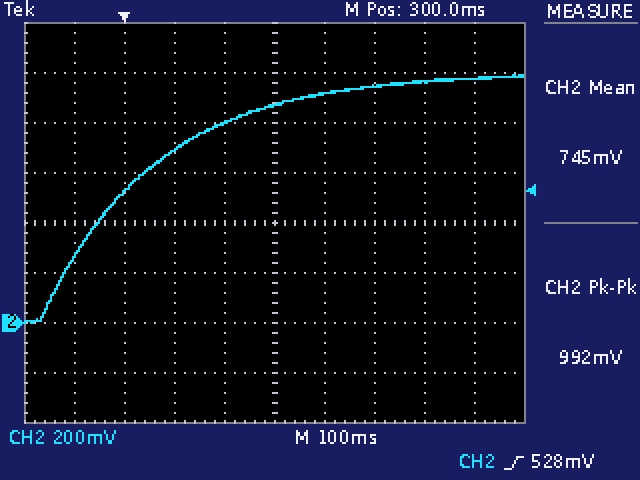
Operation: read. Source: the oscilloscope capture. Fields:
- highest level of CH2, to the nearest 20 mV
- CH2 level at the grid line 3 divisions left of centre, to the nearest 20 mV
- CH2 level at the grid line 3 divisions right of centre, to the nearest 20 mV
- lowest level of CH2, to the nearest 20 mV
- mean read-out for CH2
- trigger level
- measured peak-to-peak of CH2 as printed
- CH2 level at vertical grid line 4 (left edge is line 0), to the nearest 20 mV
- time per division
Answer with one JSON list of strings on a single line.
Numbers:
["1.00 V", "520 mV", "960 mV", "0 mV", "745 mV", "528 mV", "992 mV", "800 mV", "100 ms"]
